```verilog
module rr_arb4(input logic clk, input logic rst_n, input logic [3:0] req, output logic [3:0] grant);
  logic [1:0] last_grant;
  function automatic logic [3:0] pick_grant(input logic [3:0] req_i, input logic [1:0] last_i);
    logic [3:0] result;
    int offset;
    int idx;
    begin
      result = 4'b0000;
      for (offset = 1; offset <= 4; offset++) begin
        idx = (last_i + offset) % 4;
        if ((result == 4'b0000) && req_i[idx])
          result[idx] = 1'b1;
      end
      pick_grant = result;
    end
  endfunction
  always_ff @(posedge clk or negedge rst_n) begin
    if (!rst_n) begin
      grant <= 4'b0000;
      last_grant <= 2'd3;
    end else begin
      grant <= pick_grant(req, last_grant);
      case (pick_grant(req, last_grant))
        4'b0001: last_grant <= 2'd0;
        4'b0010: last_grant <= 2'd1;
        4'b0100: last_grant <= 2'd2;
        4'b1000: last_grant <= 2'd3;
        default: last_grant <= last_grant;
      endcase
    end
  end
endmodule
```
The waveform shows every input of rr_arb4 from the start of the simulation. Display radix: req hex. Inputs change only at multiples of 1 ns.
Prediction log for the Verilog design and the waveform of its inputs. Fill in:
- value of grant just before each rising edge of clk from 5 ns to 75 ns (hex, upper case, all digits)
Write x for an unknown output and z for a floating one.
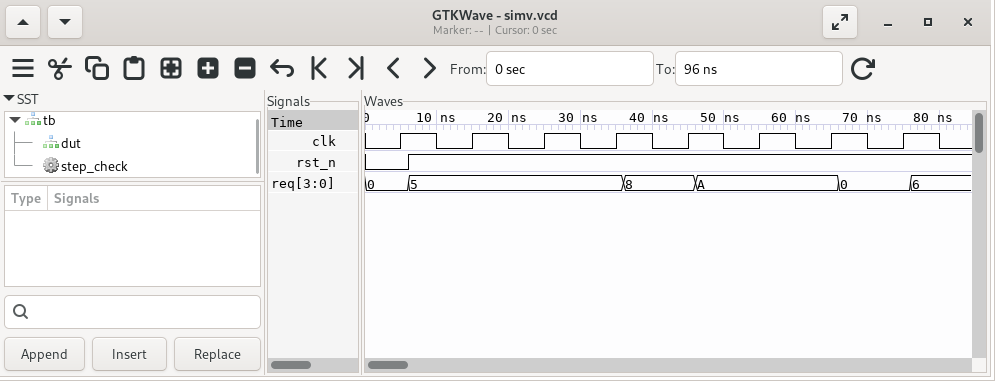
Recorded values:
0, 0, 1, 4, 1, 8, 2, 8
